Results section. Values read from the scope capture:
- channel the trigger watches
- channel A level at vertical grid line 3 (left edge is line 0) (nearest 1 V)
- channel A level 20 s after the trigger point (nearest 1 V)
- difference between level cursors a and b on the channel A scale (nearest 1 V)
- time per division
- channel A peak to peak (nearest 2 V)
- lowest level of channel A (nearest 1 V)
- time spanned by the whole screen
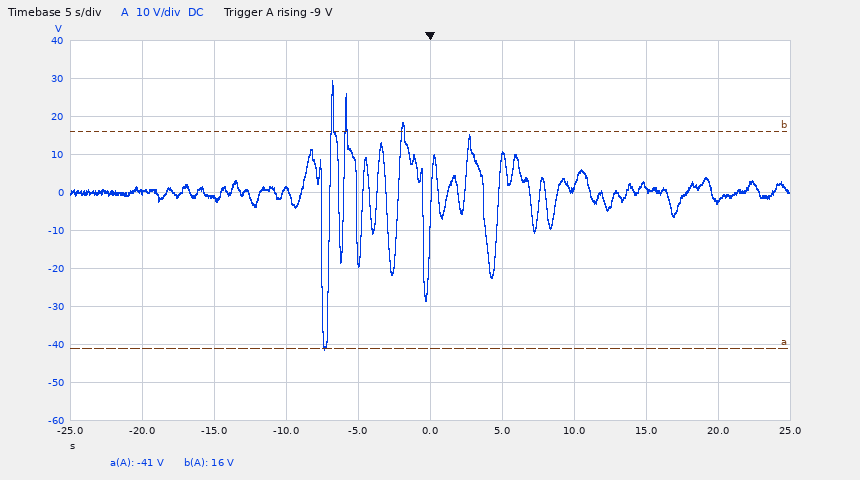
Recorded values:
channel A
1 V
-2 V
57 V
5 s
70 V
-41 V
50 s
